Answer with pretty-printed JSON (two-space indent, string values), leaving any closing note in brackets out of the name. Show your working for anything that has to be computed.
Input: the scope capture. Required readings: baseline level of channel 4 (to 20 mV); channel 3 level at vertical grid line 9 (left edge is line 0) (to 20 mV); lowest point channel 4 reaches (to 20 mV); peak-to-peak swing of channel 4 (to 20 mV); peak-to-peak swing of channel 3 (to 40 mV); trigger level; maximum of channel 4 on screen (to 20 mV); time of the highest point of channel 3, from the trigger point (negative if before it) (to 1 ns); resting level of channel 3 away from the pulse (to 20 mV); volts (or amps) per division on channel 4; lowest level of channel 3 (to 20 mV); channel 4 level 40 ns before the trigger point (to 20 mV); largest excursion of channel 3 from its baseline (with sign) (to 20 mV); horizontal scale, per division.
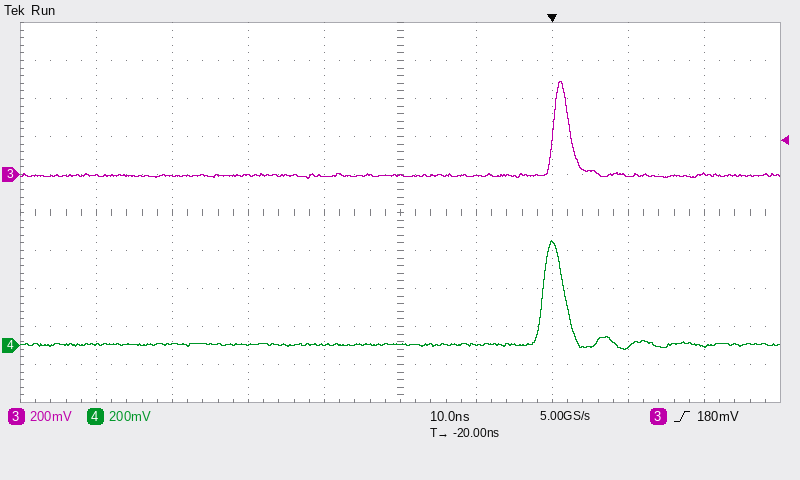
{
  "baseline level of channel 4": "0 mV",
  "channel 3 level at vertical grid line 9 (left edge is line 0)": "0 mV",
  "lowest point channel 4 reaches": "-20 mV",
  "peak-to-peak swing of channel 4": "560 mV − (-20 mV) = 580 mV",
  "peak-to-peak swing of channel 3": "520 mV",
  "trigger level": "180 mV",
  "maximum of channel 4 on screen": "560 mV",
  "time of the highest point of channel 3, from the trigger point (negative if before it)": "+1 ns",
  "resting level of channel 3 away from the pulse": "0 mV",
  "volts (or amps) per division on channel 4": "200 mV",
  "lowest level of channel 3": "-20 mV",
  "channel 4 level 40 ns before the trigger point": "0 mV",
  "largest excursion of channel 3 from its baseline (with sign)": "+500 mV",
  "horizontal scale, per division": "10 ns"
}
